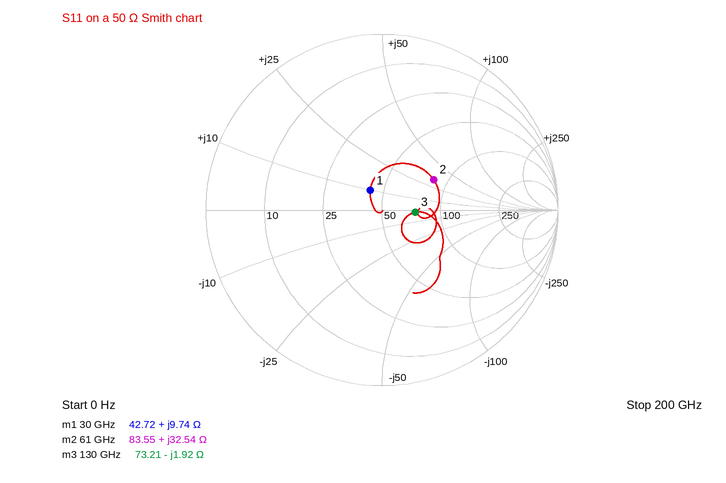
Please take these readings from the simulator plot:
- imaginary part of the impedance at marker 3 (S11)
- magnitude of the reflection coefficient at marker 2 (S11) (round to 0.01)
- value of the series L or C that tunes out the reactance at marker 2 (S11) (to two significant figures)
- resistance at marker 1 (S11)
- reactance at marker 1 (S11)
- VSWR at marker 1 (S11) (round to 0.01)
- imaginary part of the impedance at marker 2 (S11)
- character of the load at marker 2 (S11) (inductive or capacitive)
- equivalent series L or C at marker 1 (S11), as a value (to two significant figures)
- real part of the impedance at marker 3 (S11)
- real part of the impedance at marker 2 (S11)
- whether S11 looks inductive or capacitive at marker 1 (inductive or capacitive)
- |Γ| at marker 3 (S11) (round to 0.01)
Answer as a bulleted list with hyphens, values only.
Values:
- -1.92 Ω
- 0.34
- 80 fF
- 42.72 Ω
- +9.74 Ω
- 1.30
- +32.54 Ω
- inductive
- 52 pH
- 73.21 Ω
- 83.55 Ω
- inductive
- 0.19
